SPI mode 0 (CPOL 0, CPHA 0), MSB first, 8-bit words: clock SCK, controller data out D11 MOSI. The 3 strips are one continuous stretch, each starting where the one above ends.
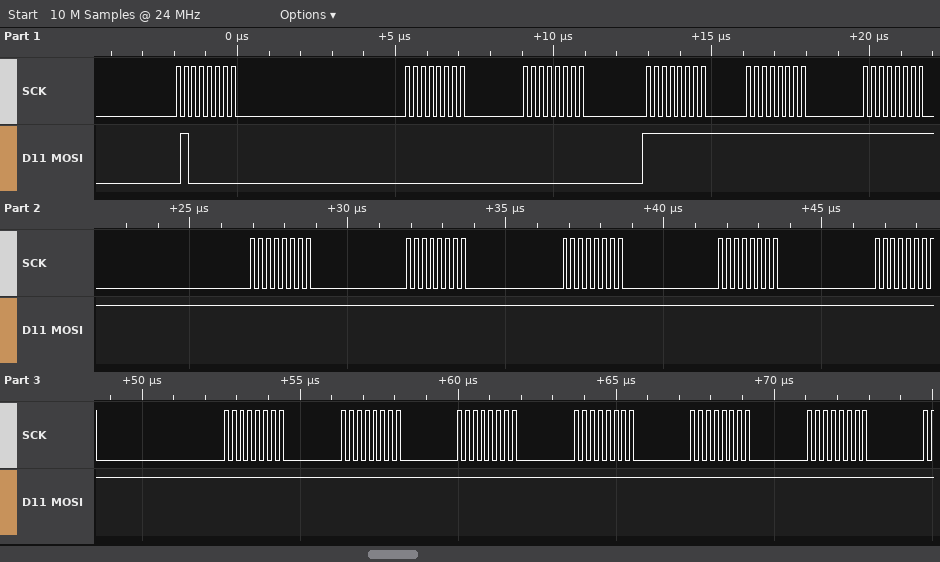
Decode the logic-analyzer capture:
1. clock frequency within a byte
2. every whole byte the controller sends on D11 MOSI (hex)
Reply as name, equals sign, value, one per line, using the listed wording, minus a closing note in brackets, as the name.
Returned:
clock frequency within a byte = 4 MHz
every whole byte the controller sends on D11 MOSI = 40 00 00 FF FF FF FF FF FF FF FF FF FF FF FF FF FF
